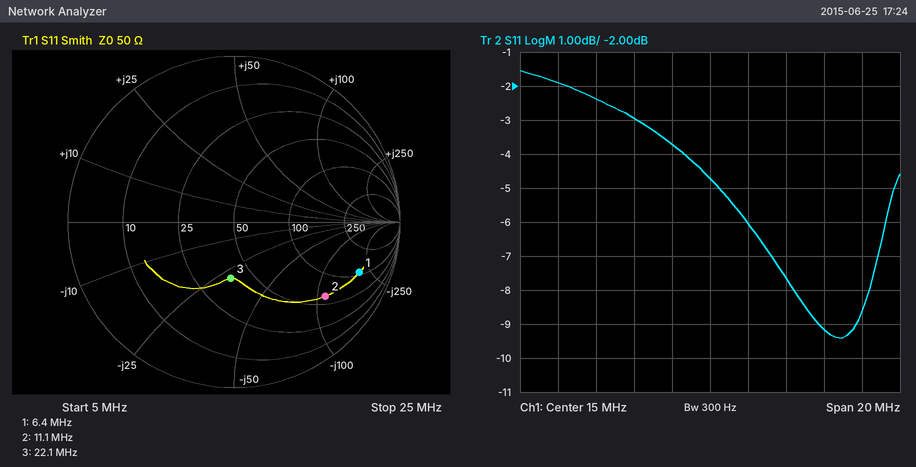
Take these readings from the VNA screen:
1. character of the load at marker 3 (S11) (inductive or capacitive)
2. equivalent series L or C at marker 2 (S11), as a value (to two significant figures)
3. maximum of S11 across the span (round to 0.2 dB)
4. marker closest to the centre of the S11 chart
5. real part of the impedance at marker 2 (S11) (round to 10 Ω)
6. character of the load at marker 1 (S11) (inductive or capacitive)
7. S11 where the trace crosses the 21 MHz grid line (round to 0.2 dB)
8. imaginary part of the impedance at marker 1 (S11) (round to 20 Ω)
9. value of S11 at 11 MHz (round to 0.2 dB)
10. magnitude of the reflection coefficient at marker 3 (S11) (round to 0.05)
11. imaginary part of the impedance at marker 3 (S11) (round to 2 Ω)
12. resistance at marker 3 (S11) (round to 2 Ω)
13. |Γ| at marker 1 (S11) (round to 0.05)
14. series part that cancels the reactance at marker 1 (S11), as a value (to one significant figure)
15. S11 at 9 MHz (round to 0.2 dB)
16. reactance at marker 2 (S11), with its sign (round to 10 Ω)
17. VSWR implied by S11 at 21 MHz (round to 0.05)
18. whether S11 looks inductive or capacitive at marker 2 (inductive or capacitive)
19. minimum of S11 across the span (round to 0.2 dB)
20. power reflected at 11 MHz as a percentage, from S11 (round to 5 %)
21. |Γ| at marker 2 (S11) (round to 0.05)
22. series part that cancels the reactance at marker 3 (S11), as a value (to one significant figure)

capacitive
130 pF
-1.6 dB
marker 3
60 Ω
capacitive
-9.2 dB
-200 Ω
-3.0 dB
0.35
-30 Ω
38 Ω
0.80
5 µH
-2.4 dB
-110 Ω
2.05
capacitive
-9.4 dB
50 %
0.70
200 nH
